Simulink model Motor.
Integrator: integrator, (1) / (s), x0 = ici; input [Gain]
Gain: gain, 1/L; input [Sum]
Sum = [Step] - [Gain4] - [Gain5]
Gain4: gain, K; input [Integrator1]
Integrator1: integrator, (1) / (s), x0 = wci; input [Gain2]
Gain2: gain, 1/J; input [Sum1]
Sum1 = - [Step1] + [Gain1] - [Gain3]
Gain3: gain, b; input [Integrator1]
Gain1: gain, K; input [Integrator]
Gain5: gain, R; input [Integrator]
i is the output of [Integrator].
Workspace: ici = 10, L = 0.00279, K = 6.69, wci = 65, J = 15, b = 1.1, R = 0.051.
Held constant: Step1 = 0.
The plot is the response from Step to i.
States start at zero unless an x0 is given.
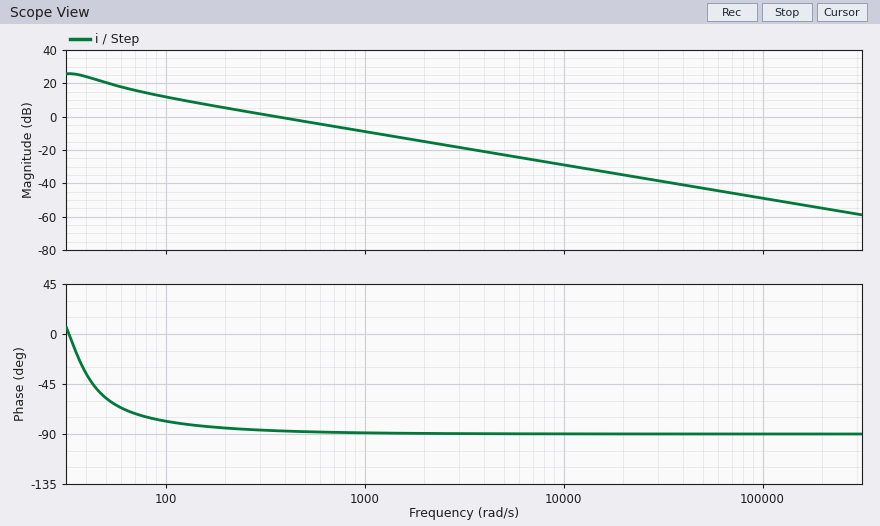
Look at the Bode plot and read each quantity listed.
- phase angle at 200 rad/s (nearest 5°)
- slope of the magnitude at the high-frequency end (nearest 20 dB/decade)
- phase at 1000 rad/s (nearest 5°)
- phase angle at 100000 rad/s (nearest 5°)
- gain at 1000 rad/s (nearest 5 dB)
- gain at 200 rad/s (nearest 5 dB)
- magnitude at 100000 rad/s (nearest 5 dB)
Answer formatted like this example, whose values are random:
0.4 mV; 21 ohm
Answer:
-85°; -20 dB/decade; -90°; -90°; -10 dB; 5 dB; -50 dB
